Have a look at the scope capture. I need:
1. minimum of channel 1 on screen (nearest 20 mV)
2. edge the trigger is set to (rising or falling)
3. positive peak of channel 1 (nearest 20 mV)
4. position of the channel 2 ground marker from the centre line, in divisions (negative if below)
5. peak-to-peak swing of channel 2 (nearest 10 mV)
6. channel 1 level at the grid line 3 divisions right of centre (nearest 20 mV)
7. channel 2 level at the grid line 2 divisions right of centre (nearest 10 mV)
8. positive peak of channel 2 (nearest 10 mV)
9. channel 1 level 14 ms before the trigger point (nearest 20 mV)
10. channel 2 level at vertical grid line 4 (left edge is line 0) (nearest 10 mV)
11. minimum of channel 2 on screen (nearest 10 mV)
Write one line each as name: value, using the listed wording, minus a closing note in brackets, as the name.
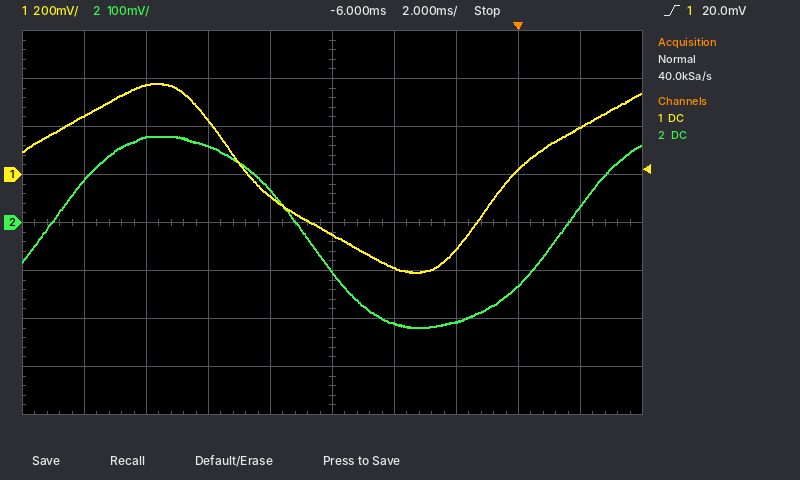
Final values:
minimum of channel 1 on screen: -400 mV
edge the trigger is set to: rising
positive peak of channel 1: 380 mV
position of the channel 2 ground marker from the centre line, in divisions: 0.0 div
peak-to-peak swing of channel 2: 400 mV
channel 1 level at the grid line 3 divisions right of centre: 20 mV
channel 2 level at the grid line 2 divisions right of centre: -210 mV
positive peak of channel 2: 180 mV
channel 1 level 14 ms before the trigger point: 240 mV
channel 2 level at vertical grid line 4 (left edge is line 0): 70 mV
minimum of channel 2 on screen: -220 mV
